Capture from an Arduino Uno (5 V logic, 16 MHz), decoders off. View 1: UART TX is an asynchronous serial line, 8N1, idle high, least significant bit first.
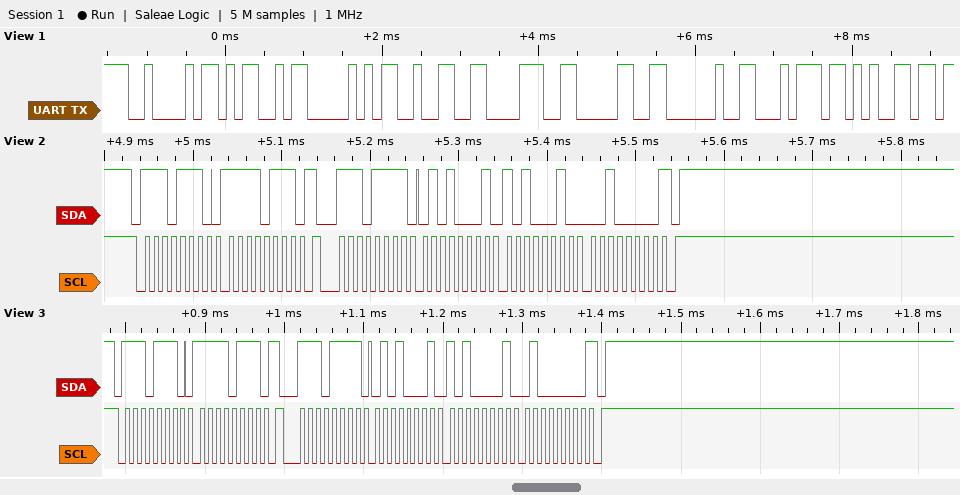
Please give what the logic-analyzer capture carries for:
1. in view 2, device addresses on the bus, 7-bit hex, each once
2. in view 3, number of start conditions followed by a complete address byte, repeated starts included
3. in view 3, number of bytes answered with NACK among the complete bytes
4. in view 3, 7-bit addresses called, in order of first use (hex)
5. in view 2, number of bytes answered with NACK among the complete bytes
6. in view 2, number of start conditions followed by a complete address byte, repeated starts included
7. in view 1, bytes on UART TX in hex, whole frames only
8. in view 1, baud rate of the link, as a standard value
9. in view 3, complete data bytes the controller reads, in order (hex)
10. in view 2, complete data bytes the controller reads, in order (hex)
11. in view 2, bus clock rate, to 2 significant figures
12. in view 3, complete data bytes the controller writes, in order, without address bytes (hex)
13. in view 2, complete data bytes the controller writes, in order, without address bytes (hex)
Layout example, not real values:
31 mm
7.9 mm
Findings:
0x77
2
1
0x77
1
2
42 4D 50 32 38 30 20 74 65
9600 baud
51 A1 40
51 A2 20
100 kHz
F7
F7
